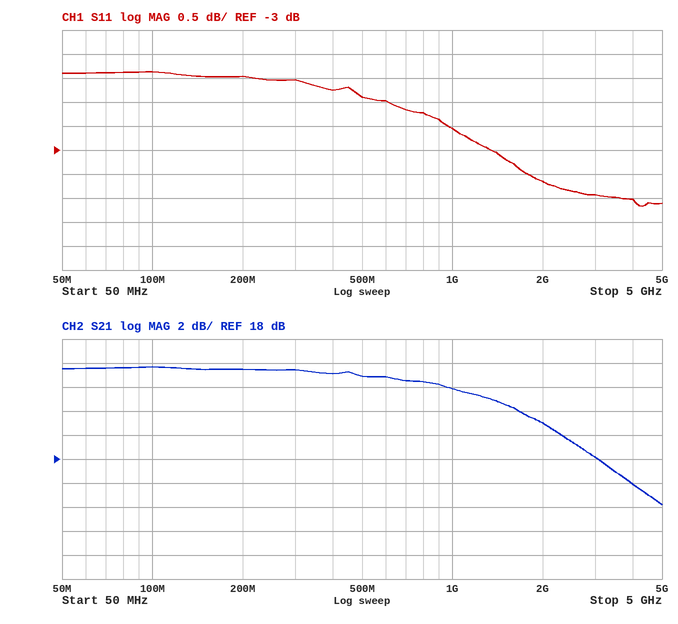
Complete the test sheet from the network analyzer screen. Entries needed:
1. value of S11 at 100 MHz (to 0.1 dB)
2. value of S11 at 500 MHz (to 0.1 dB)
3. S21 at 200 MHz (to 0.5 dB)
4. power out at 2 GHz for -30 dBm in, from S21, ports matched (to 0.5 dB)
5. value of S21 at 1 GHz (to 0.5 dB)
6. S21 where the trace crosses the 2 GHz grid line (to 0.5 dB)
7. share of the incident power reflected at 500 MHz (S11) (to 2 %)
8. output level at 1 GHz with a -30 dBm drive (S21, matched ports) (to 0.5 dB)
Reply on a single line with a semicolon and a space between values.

-1.4 dB; -1.9 dB; 25.5 dB; -9.0 dBm; 24.0 dB; 21.0 dB; 64 %; -6.0 dBm
